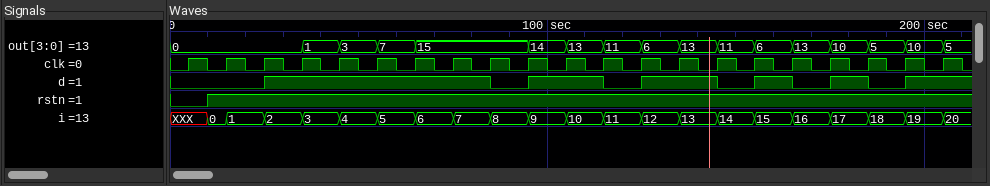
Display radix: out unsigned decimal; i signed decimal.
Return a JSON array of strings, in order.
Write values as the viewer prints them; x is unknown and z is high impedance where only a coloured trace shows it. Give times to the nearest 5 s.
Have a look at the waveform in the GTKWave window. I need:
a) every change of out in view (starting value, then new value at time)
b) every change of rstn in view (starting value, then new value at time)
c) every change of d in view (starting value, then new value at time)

["0, 1 at 35 s, 3 at 45 s, 7 at 55 s, 15 at 65 s, 14 at 95 s, 13 at 105 s, 11 at 115 s, 6 at 125 s, 13 at 135 s, 11 at 145 s, 6 at 155 s, 13 at 165 s, 10 at 175 s, 5 at 185 s, 10 at 195 s, 5 at 205 s", "0, 1 at 10 s", "0, 1 at 25 s, 0 at 85 s, 1 at 95 s, 0 at 115 s, 1 at 125 s, 0 at 145 s, 1 at 155 s, 0 at 165 s, 1 at 175 s, 0 at 185 s, 1 at 195 s"]
